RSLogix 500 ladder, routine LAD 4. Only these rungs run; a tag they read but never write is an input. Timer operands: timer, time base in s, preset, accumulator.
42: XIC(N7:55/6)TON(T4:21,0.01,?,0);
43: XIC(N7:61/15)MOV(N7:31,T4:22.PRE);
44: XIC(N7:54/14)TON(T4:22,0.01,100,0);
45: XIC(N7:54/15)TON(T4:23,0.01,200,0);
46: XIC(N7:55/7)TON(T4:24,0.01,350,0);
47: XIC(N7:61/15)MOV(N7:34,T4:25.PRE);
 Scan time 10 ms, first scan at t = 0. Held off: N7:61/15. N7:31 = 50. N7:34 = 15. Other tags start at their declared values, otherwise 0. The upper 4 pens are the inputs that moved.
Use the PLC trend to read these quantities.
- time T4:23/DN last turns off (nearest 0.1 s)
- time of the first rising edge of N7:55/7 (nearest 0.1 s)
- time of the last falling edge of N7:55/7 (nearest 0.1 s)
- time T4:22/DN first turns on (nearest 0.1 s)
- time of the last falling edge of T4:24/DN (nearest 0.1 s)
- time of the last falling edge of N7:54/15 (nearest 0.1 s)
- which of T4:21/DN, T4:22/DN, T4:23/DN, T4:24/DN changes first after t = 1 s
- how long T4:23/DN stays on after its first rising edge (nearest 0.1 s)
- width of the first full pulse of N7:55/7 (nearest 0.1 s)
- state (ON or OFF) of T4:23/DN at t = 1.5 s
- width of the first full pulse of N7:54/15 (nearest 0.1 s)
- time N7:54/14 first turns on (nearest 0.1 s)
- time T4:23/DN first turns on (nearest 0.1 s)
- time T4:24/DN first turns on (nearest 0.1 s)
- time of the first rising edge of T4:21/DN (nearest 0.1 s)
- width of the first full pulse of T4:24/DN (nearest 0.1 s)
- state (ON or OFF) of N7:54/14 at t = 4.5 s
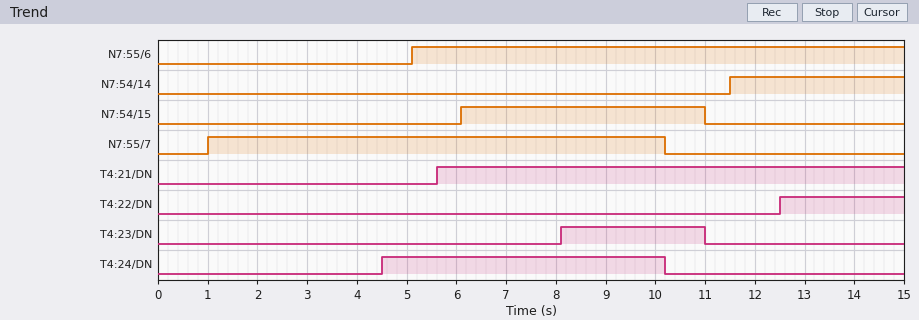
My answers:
11.0 s
1.0 s
10.2 s
12.5 s
10.2 s
11.0 s
T4:24/DN
2.9 s
9.2 s
OFF
4.9 s
11.5 s
8.1 s
4.5 s
5.6 s
5.7 s
OFF
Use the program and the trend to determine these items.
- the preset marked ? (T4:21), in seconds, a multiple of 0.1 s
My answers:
0.5 s
